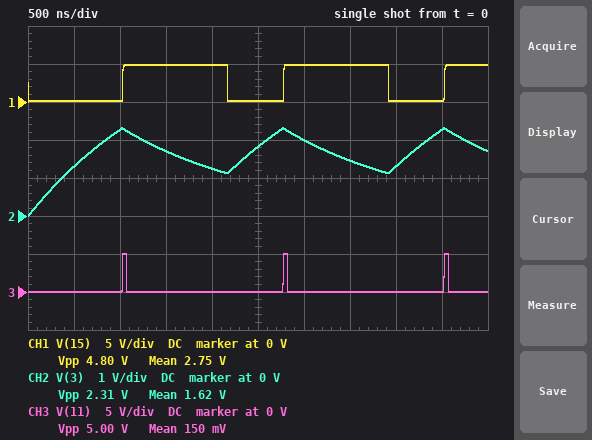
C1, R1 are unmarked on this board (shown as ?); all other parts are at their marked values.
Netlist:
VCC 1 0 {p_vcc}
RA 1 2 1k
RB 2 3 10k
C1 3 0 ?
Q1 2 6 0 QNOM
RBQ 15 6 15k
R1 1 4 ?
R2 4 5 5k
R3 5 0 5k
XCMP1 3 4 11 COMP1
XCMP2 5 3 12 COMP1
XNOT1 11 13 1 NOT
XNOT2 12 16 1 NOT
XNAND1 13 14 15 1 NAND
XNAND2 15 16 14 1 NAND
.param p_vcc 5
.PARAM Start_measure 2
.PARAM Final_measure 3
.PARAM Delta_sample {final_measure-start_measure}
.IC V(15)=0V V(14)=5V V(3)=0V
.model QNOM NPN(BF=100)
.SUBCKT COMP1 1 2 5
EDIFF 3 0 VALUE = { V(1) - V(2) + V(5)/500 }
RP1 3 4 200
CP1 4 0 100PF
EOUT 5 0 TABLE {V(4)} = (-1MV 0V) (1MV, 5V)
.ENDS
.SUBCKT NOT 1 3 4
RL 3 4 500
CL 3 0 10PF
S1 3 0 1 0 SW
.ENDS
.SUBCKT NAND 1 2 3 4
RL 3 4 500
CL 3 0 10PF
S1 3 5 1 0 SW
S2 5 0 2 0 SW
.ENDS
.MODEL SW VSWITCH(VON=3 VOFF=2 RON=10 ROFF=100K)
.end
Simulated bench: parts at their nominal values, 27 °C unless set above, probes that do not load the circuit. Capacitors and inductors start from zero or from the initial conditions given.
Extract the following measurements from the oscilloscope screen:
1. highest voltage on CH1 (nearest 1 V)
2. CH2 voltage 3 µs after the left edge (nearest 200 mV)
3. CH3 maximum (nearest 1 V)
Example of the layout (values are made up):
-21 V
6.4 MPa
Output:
5 V
2.0 V
5 V
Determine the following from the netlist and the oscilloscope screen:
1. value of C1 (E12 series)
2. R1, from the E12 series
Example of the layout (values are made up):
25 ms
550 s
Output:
150 pF
12 kΩ
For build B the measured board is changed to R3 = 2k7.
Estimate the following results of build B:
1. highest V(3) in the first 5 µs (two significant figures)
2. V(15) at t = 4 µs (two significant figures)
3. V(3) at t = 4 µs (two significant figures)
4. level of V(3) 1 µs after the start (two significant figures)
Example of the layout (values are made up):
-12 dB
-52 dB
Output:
2.0 V
4.8 V
1.2 V
1.8 V
